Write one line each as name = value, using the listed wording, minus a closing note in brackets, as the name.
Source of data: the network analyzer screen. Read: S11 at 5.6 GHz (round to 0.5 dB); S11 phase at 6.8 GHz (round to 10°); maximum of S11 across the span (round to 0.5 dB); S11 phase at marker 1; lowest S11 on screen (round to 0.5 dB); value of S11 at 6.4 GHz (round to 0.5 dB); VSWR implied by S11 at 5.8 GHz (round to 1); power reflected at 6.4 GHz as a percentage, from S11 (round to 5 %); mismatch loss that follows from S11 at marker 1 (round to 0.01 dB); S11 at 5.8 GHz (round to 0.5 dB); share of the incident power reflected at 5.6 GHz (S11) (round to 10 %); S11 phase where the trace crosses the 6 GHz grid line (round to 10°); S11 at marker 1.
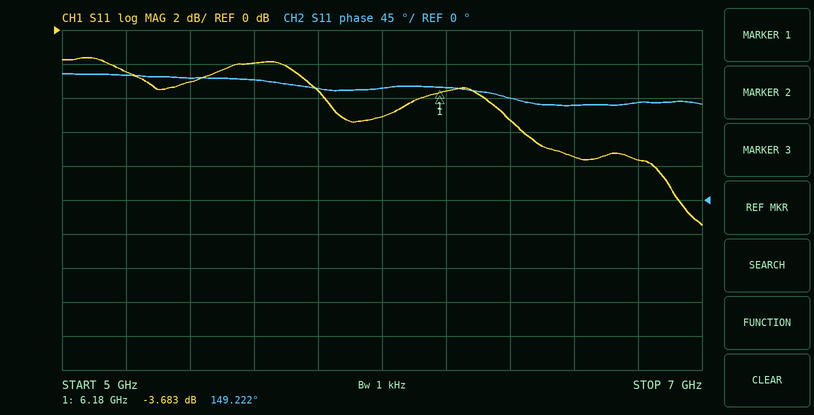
S11 at 5.6 GHz = -2.0 dB
S11 phase at 6.8 GHz = 130°
maximum of S11 across the span = -1.5 dB
S11 phase at marker 1 = 149.222°
lowest S11 on screen = -11.5 dB
value of S11 at 6.4 GHz = -5.5 dB
VSWR implied by S11 at 5.8 GHz = 5
power reflected at 6.4 GHz as a percentage, from S11 = 30 %
mismatch loss that follows from S11 at marker 1 = 2.43 dB
S11 at 5.8 GHz = -3.5 dB
share of the incident power reflected at 5.6 GHz (S11) = 60 %
S11 phase where the trace crosses the 6 GHz grid line = 150°
S11 at marker 1 = -3.683 dB
